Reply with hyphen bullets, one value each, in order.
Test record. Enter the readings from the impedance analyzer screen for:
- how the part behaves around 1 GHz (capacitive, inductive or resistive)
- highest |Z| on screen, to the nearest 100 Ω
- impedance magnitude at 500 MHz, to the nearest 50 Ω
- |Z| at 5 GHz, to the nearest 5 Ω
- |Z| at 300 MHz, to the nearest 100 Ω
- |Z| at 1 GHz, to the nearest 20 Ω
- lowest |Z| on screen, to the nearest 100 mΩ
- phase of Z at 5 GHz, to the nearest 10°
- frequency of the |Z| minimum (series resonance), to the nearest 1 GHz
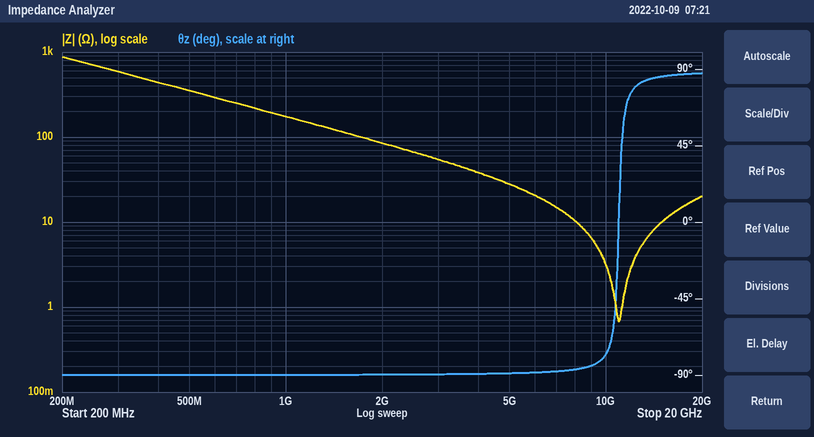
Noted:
- capacitive
- 900 Ω
- 350 Ω
- 30 Ω
- 600 Ω
- 180 Ω
- 700 mΩ
- -90°
- 11 GHz
